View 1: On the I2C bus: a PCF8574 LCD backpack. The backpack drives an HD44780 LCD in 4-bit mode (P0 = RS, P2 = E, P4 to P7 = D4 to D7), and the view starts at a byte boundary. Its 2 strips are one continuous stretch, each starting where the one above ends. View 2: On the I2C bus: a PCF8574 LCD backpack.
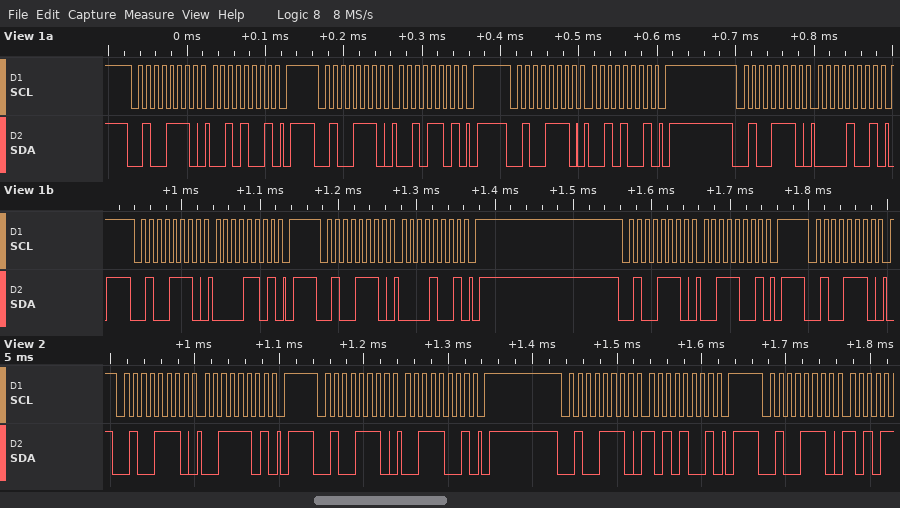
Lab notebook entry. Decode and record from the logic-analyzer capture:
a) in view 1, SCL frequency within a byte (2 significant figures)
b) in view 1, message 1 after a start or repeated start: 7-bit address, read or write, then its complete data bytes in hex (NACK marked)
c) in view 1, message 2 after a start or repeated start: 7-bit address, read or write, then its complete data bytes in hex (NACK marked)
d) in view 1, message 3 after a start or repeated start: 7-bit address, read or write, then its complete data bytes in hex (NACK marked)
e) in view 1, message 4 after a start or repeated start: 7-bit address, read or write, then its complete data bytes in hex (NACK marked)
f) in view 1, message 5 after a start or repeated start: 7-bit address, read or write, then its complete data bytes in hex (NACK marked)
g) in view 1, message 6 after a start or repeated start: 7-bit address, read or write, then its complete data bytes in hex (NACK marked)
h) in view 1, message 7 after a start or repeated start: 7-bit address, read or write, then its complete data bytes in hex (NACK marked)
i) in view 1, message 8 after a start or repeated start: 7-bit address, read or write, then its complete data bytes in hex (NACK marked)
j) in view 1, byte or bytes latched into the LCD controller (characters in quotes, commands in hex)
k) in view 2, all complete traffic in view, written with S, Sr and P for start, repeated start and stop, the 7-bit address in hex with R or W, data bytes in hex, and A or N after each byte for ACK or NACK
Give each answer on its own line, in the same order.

100 kHz
0x27 write: 29
0x27 write: 2D
0x27 write: 29
0x27 write: 09
0x27 write: 0D
0x27 write: 09
0x27 write: 39
0x27 write
' '
S 27W A 3D A P S 27W A 39 A P S 27W A A9 A P S 27W A
